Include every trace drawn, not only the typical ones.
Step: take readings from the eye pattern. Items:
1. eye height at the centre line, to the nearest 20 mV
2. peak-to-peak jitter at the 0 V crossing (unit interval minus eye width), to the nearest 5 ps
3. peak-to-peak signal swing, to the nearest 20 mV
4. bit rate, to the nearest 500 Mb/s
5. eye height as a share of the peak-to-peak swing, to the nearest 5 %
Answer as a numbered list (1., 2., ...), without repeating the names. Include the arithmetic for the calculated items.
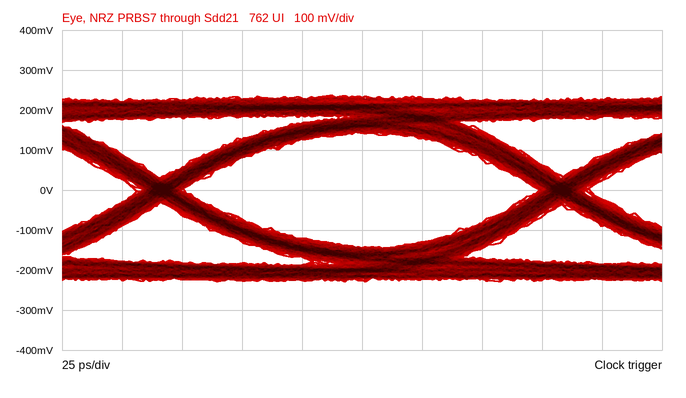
1. 280 mV
2. 20 ps
3. 460 mV
4. 6.0 Gb/s
5. 280 mV / 460 mV ≈ 60.9 %, so 60 % to the nearest 5 %
